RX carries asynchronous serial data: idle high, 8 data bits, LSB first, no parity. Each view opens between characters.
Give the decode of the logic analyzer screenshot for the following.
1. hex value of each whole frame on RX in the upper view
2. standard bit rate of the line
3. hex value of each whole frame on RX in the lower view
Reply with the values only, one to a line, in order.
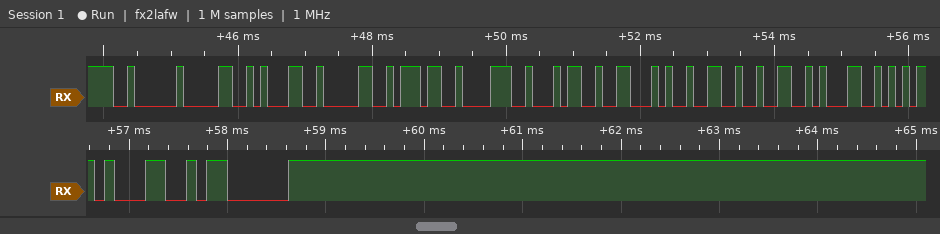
02, 30, 31, 30, 37, 38, 34, 46, 32, 32, 31
9600 baud
31, 03
